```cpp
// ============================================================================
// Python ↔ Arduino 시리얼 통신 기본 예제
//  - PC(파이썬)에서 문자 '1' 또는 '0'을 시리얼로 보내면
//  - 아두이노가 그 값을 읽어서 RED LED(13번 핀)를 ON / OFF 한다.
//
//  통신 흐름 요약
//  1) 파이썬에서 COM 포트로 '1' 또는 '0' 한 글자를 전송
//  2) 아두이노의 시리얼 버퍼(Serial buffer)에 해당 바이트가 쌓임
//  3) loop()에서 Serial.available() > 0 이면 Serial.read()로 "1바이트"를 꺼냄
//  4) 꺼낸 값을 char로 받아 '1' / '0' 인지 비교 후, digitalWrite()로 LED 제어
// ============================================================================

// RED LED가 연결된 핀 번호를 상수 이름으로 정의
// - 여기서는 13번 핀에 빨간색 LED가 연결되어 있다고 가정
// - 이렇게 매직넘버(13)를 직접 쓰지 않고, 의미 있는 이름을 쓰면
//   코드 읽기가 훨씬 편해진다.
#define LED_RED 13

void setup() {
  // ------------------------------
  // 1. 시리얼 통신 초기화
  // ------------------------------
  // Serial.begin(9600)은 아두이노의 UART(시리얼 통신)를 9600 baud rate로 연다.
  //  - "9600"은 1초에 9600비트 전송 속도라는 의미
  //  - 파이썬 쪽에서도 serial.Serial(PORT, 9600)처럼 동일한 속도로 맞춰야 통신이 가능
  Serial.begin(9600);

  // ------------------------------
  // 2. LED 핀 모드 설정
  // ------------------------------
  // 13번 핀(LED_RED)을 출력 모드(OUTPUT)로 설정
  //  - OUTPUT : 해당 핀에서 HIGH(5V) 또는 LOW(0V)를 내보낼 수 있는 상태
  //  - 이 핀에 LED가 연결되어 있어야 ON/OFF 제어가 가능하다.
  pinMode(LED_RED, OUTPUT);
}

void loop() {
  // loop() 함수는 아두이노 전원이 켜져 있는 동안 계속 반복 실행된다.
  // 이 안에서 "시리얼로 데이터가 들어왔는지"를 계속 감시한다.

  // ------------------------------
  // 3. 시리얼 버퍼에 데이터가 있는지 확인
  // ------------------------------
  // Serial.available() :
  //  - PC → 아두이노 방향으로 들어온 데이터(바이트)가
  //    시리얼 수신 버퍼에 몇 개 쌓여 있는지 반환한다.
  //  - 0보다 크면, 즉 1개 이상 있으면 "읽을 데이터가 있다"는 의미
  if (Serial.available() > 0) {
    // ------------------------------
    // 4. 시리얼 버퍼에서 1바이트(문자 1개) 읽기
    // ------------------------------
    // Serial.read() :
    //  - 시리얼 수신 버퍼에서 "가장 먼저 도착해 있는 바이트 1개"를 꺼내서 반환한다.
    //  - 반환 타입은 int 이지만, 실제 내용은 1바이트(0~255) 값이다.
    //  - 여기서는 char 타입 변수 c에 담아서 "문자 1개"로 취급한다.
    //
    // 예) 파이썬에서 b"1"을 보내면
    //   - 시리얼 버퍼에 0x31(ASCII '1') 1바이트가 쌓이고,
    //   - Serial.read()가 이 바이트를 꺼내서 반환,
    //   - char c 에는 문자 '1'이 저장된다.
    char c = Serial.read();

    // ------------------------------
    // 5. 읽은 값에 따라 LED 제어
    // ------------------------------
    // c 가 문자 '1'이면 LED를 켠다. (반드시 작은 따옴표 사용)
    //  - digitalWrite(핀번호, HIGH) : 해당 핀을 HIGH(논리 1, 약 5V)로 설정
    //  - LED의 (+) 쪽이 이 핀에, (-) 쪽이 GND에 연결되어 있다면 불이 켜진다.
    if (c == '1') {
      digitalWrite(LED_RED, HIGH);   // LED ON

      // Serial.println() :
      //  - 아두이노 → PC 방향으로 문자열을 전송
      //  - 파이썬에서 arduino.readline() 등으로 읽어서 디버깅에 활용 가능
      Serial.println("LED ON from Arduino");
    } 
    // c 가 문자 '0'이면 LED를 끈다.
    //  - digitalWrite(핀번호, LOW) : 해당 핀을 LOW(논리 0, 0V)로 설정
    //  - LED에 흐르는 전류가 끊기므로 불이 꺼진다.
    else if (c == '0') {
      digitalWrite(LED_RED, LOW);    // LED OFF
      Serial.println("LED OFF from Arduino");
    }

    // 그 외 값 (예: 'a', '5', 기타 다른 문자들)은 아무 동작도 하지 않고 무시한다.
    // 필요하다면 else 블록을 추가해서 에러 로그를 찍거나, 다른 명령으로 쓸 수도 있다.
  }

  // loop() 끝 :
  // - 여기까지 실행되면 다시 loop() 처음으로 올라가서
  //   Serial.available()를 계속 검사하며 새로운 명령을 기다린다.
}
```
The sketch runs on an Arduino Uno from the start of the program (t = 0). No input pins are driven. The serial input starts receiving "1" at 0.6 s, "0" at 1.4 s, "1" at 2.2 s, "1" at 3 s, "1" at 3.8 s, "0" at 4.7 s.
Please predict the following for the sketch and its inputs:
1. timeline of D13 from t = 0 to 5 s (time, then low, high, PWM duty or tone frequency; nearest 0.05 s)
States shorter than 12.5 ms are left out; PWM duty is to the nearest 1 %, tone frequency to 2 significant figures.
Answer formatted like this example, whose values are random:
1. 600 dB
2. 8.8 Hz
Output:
1. 0 s low; 0.6 s high; 1.4 s low; 2.2 s high; 4.7 s low
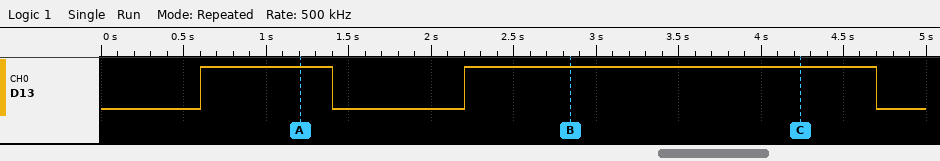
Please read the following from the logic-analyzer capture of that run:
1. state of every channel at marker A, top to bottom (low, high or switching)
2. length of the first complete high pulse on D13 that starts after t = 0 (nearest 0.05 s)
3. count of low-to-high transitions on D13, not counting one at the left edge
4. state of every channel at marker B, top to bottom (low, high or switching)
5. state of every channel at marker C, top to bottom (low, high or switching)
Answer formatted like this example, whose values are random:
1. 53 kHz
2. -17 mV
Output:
1. D13 high
2. 0.80 s
3. 2
4. D13 high
5. D13 high
